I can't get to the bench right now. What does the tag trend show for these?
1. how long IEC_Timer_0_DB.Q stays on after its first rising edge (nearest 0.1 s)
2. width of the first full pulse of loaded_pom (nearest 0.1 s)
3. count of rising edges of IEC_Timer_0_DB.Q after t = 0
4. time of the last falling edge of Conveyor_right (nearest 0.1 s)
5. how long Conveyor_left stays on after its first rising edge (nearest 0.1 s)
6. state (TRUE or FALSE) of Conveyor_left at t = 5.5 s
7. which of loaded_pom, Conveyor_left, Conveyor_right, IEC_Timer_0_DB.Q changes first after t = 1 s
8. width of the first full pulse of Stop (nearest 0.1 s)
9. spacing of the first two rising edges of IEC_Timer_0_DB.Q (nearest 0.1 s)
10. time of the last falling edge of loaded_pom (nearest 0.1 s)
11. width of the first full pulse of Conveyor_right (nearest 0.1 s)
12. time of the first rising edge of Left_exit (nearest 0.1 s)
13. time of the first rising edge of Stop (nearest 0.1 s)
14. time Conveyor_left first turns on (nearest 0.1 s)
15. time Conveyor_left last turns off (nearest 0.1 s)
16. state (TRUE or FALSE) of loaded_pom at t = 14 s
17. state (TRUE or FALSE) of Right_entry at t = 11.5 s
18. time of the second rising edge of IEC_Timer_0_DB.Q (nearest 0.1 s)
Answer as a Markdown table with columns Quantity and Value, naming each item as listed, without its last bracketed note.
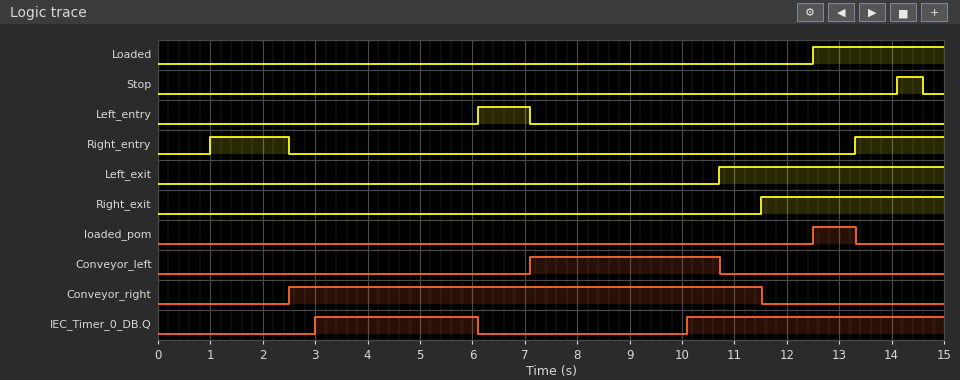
| Quantity | Value |
|---|---|
| how long IEC_Timer_0_DB.Q stays on after its first rising edge | 3.1 s |
| width of the first full pulse of loaded_pom | 0.8 s |
| count of rising edges of IEC_Timer_0_DB.Q after t = 0 | 2 |
| time of the last falling edge of Conveyor_right | 11.5 s |
| how long Conveyor_left stays on after its first rising edge | 3.6 s |
| state (TRUE or FALSE) of Conveyor_left at t = 5.5 s | FALSE |
| which of loaded_pom, Conveyor_left, Conveyor_right, IEC_Timer_0_DB.Q changes first after t = 1 s | Conveyor_right |
| width of the first full pulse of Stop | 0.5 s |
| spacing of the first two rising edges of IEC_Timer_0_DB.Q | 7.1 s |
| time of the last falling edge of loaded_pom | 13.3 s |
| width of the first full pulse of Conveyor_right | 9.0 s |
| time of the first rising edge of Left_exit | 10.7 s |
| time of the first rising edge of Stop | 14.1 s |
| time Conveyor_left first turns on | 7.1 s |
| time Conveyor_left last turns off | 10.7 s |
| state (TRUE or FALSE) of loaded_pom at t = 14 s | FALSE |
| state (TRUE or FALSE) of Right_entry at t = 11.5 s | FALSE |
| time of the second rising edge of IEC_Timer_0_DB.Q | 10.1 s |
